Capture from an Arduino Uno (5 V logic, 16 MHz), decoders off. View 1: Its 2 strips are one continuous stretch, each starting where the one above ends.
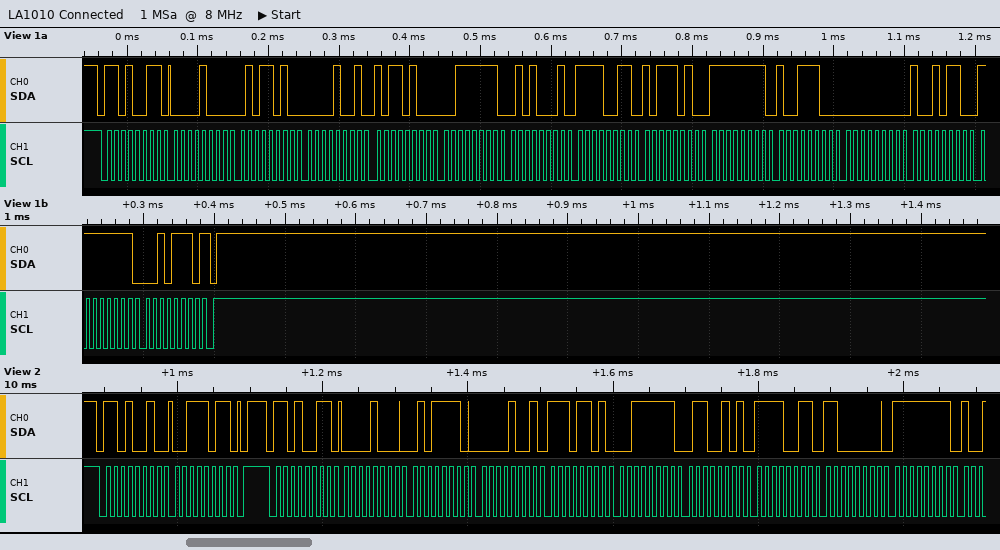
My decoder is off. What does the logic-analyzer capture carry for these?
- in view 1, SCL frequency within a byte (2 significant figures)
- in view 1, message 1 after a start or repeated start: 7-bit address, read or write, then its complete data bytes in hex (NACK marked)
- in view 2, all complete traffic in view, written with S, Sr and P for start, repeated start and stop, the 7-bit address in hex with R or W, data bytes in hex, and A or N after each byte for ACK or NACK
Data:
100 kHz
0x69 read: 08 5A 09 B4 3F 51 F3 BA FF 9C 00 96 FF 2E NACK
S 69W A 3B A P S 69R A 08 A 5E A 09 A ED A 3F A 65 A F3 A C0 A FF A
